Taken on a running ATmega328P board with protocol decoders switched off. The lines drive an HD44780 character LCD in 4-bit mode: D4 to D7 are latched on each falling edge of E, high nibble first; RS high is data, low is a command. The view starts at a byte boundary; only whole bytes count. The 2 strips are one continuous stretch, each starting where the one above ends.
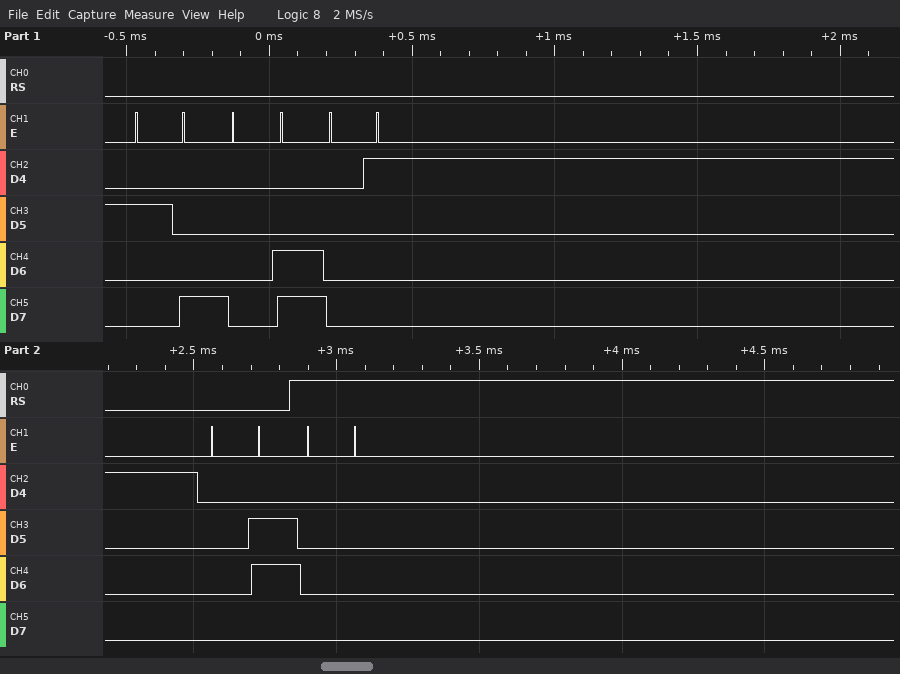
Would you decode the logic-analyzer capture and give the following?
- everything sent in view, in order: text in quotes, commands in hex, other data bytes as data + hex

0x28 0x0C 0x01 0x06 data 00
